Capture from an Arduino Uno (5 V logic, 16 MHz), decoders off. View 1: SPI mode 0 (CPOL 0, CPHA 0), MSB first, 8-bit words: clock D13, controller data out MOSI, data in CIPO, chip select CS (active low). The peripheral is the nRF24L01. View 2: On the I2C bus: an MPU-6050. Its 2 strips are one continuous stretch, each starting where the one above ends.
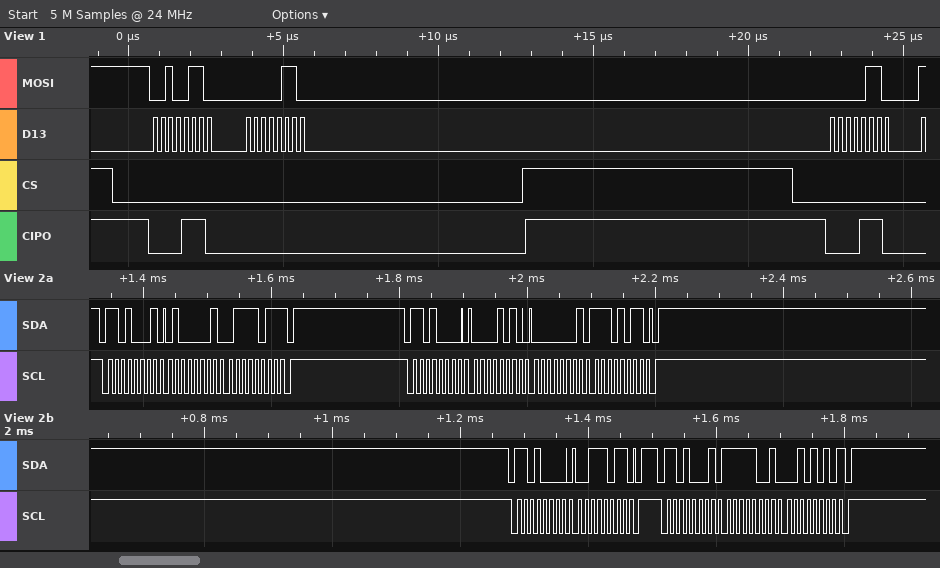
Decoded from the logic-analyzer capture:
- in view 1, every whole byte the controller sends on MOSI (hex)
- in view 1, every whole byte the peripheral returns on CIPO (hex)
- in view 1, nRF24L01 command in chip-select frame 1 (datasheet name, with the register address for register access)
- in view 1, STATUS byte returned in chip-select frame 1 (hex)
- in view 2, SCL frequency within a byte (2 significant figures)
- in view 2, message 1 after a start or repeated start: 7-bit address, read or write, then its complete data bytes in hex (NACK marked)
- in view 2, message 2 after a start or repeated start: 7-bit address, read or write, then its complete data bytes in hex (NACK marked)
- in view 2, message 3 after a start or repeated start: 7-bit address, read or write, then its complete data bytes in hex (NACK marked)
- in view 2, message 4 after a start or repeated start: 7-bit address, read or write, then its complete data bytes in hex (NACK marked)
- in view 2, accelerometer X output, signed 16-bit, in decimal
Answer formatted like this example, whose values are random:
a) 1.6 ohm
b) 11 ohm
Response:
a) 26 06 06
b) 0E 00 0E
c) W_REGISTER 0x06
d) 0x0E
e) 100 kHz
f) 0x68 read: 41 7B NACK
g) 0x68 write: 0A 01 EB
h) 0x68 write: 3B
i) 0x68 read: F9 2A NACK
j) -1750
